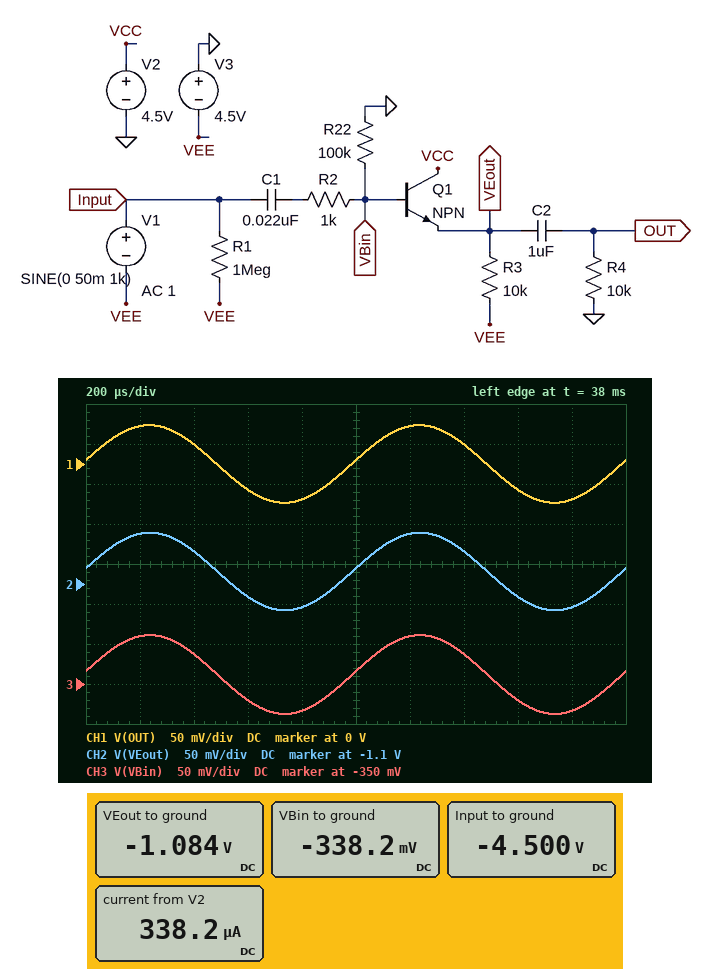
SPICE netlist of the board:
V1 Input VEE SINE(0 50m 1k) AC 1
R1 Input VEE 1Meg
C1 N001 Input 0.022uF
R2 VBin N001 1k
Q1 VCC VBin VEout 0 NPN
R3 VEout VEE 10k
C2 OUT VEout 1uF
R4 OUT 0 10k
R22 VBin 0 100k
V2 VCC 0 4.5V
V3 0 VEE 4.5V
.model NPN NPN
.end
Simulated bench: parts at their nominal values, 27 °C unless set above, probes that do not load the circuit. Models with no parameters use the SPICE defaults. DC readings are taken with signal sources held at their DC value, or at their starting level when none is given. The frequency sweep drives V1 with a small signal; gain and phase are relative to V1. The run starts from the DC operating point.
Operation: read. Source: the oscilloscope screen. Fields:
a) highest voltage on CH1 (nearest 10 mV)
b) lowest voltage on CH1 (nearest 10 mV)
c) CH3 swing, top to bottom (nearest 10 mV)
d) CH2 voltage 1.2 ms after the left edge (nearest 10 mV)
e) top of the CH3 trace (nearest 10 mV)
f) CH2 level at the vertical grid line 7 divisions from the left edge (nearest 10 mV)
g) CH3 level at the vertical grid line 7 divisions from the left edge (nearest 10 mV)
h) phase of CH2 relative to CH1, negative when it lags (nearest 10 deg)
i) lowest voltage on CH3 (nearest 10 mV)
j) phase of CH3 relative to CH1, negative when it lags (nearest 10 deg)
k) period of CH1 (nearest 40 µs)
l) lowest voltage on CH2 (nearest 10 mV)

50 mV
-50 mV
100 mV
-1.04 V
-290 mV
-1.06 V
-310 mV
0 deg
-390 mV
0 deg
1.00 ms
-1.13 V
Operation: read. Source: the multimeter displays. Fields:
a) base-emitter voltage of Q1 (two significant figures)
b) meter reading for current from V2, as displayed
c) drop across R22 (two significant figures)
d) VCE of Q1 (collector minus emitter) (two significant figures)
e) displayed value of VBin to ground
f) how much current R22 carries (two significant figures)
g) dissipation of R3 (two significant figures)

750 mV
338.2 µA
340 mV
5.6 V
-338.2 mV
3.4 µA
1.2 mW
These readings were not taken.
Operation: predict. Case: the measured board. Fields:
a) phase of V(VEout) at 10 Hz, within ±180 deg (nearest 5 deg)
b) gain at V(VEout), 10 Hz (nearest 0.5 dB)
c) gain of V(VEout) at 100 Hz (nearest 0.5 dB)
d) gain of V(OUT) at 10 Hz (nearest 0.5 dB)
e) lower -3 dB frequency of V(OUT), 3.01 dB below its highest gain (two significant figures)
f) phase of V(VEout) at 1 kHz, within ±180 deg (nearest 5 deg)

80 deg
-18.5 dB
-2.5 dB
-24.0 dB
89 Hz
5 deg
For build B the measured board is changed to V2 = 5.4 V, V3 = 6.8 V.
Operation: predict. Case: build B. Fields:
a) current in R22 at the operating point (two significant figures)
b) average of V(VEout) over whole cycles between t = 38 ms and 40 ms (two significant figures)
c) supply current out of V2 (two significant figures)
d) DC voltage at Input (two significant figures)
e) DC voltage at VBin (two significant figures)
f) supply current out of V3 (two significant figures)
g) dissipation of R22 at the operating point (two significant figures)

5.4 µA
-1.3 V
540 µA
-6.8 V
-540 mV
550 µA
3.0 µW
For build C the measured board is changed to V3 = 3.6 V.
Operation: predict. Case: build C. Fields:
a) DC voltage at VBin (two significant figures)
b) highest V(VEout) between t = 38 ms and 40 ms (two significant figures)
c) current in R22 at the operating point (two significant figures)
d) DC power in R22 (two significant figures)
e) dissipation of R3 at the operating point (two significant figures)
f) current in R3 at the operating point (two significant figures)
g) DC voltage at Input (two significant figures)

-260 mV
-950 mV
2.6 µA
660 nW
680 µW
260 µA
-3.6 V
